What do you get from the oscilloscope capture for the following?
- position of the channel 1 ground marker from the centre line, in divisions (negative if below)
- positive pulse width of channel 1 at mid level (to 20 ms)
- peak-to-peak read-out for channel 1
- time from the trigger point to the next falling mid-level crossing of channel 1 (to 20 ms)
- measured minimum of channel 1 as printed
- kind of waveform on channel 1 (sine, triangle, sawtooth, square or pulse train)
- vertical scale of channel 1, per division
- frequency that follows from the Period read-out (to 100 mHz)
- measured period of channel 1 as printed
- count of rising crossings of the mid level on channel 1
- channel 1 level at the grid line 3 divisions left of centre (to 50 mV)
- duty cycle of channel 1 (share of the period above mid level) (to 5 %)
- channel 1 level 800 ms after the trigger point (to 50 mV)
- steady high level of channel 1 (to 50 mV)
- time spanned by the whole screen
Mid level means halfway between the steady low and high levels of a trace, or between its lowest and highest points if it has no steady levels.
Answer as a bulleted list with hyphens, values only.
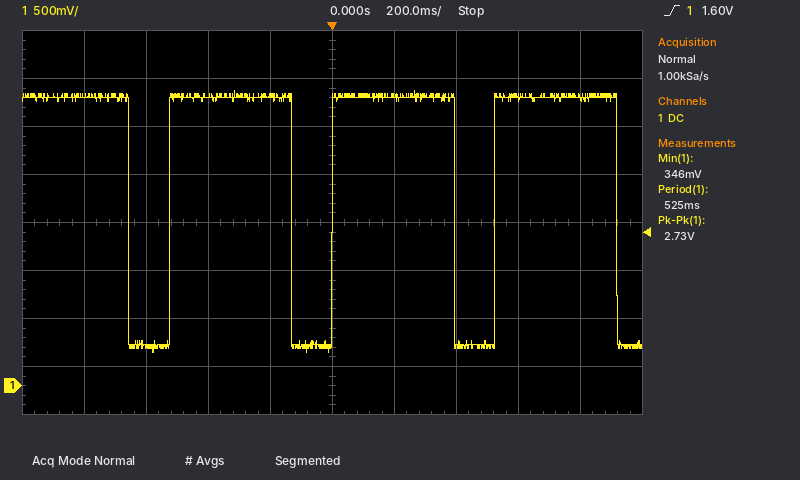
- -3.4 div
- 400 ms
- 2.73 V
- 400 ms
- 346 mV
- pulse train
- 500 mV
- 1.9 Hz
- 525 ms
- 3
- 400 mV
- 75 %
- 3.00 V
- 3.00 V
- 2 s
